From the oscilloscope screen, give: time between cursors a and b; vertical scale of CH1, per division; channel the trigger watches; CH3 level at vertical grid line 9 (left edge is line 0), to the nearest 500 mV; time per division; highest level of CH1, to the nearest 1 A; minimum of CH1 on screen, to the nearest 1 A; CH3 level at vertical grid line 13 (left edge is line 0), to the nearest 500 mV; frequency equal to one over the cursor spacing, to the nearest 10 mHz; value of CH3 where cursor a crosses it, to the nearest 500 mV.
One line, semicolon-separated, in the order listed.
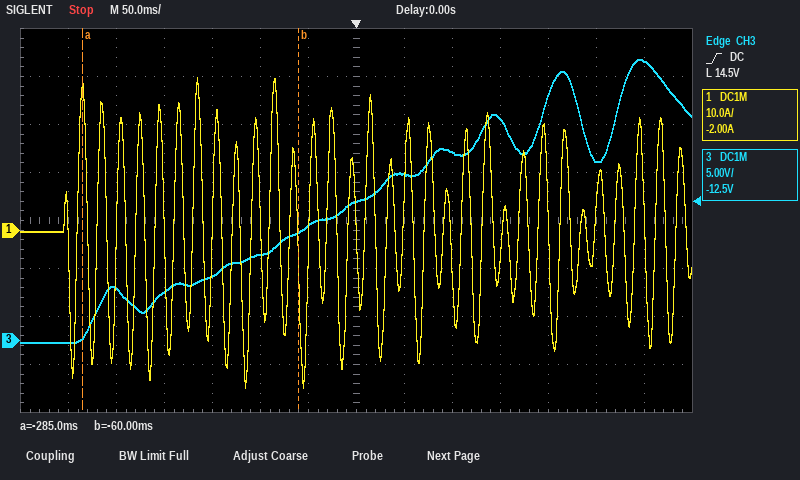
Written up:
225 ms; 10 A; CH3; 19.5 V; 50 ms; 32 A; -33 A; 29.0 V; 4.44 Hz; 500 mV
